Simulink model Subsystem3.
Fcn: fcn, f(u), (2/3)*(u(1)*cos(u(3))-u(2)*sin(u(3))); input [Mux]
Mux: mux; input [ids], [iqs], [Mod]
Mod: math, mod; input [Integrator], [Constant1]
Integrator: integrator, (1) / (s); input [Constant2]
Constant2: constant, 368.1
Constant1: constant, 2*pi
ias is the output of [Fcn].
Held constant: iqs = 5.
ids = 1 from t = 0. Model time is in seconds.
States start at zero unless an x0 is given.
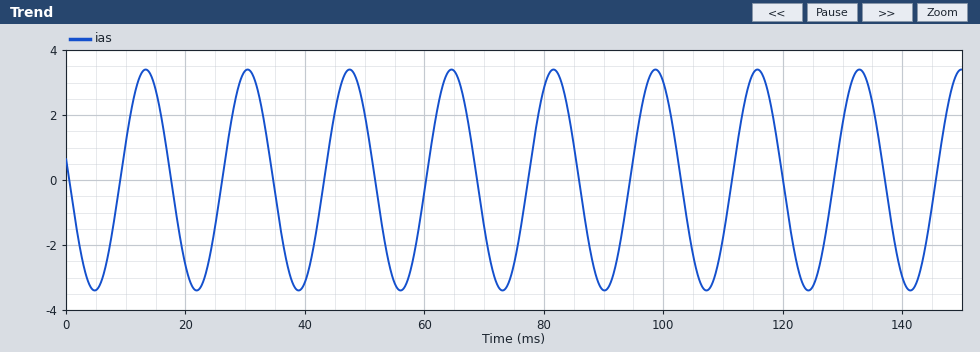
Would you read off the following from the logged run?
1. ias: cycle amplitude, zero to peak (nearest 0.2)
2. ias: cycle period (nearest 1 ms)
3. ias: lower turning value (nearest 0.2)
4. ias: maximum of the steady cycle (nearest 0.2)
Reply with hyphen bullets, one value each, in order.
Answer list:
- 3.4
- 17 ms
- -3.4
- 3.4
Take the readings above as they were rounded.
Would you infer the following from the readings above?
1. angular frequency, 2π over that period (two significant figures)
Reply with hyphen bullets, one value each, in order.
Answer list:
- 0.37 rad/ms
